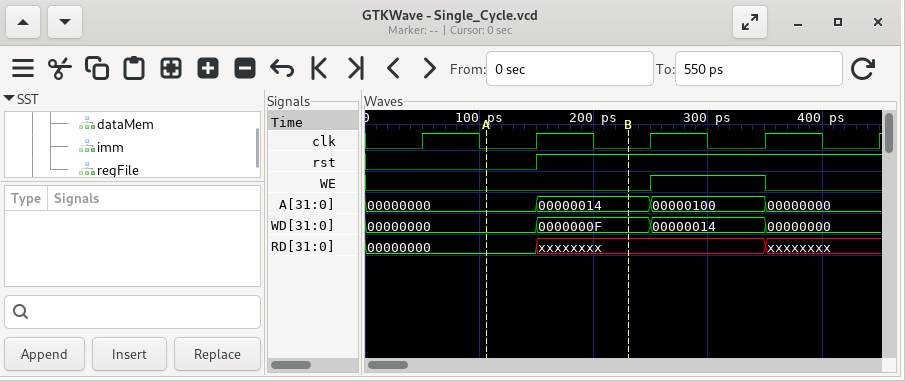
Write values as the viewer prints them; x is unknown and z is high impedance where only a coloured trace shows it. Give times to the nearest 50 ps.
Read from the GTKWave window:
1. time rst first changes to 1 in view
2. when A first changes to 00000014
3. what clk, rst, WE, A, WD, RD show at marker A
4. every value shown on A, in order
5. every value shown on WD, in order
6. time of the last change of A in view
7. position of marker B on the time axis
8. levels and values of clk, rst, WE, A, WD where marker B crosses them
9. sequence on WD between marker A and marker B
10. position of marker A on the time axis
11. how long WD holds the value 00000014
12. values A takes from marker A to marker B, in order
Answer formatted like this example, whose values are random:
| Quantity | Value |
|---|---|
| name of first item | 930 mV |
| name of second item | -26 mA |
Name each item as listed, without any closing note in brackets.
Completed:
| Quantity | Value |
|---|---|
| time rst first changes to 1 in view | 150 ps |
| when A first changes to 00000014 | 150 ps |
| what clk, rst, WE, A, WD, RD show at marker A | clk=0, rst=0, WE=0, A=00000000, WD=00000000, RD=00000000 |
| every value shown on A, in order | 00000000, 00000014, 00000100, 00000000 |
| every value shown on WD, in order | 00000000, 0000000F, 00000014, 00000000 |
| time of the last change of A in view | 350 ps |
| position of marker B on the time axis | 250 ps |
| levels and values of clk, rst, WE, A, WD where marker B crosses them | clk=0, rst=1, WE=0, A=00000014, WD=0000000F |
| sequence on WD between marker A and marker B | 00000000, 0000000F |
| position of marker A on the time axis | 100 ps |
| how long WD holds the value 00000014 | 100 ps |
| values A takes from marker A to marker B, in order | 00000000, 00000014 |
